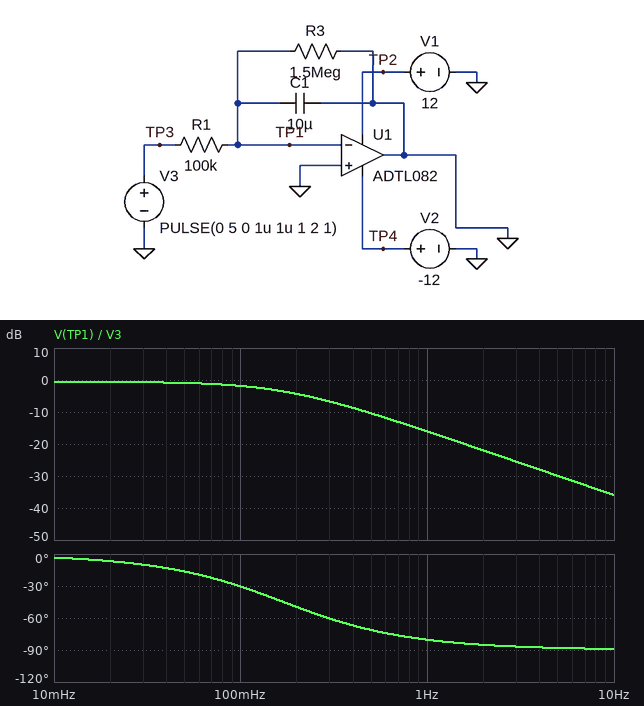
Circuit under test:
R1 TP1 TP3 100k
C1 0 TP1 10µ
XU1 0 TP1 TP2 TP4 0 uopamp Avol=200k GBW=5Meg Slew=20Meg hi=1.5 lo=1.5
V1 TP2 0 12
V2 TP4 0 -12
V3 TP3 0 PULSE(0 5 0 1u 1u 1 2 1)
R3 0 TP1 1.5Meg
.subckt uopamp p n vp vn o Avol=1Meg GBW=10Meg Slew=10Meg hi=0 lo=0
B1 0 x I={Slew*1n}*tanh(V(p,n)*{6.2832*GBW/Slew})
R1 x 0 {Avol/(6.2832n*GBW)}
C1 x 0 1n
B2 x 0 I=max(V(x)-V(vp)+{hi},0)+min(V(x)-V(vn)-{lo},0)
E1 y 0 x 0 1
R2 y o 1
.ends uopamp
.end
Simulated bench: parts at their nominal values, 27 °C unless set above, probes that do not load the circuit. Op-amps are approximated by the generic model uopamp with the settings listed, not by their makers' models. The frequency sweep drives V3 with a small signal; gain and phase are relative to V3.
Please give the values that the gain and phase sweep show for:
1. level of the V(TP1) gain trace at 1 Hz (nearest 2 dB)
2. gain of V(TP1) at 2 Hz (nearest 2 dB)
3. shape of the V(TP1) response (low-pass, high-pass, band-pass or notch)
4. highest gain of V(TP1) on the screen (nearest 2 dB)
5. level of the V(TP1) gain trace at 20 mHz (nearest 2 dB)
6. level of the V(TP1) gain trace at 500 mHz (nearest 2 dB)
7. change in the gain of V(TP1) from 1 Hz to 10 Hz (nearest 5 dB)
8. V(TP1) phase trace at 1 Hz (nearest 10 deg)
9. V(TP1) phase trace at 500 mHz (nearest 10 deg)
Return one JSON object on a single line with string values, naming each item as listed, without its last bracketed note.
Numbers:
{"level of the V(TP1) gain trace at 1 Hz": "-16 dB", "gain of V(TP1) at 2 Hz": "-22 dB", "shape of the V(TP1) response": "low-pass", "highest gain of V(TP1) on the screen": "0 dB", "level of the V(TP1) gain trace at 20 mHz": "0 dB", "level of the V(TP1) gain trace at 500 mHz": "-10 dB", "change in the gain of V(TP1) from 1 Hz to 10 Hz": "-20 dB", "V(TP1) phase trace at 1 Hz": "-80 deg", "V(TP1) phase trace at 500 mHz": "-70 deg"}
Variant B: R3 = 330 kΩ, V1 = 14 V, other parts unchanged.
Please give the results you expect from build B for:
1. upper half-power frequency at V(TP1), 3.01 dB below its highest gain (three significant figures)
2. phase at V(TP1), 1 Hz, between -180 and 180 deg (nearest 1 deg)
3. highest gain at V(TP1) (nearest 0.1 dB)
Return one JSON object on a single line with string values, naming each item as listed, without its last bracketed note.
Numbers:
{"upper half-power frequency at V(TP1), 3.01 dB below its highest gain": "207 mHz", "phase at V(TP1), 1 Hz, between -180 and 180 deg": "-78 deg", "highest gain at V(TP1)": "-2.3 dB"}
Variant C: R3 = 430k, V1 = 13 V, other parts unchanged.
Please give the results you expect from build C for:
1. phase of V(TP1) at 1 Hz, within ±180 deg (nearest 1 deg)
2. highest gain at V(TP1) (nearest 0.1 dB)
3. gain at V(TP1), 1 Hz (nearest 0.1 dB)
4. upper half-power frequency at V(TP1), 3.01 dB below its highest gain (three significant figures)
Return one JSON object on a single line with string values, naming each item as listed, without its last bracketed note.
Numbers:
{"phase of V(TP1) at 1 Hz, within ±180 deg": "-79 deg", "highest gain at V(TP1)": "-1.8 dB", "gain at V(TP1), 1 Hz": "-16.1 dB", "upper half-power frequency at V(TP1), 3.01 dB below its highest gain": "196 mHz"}
